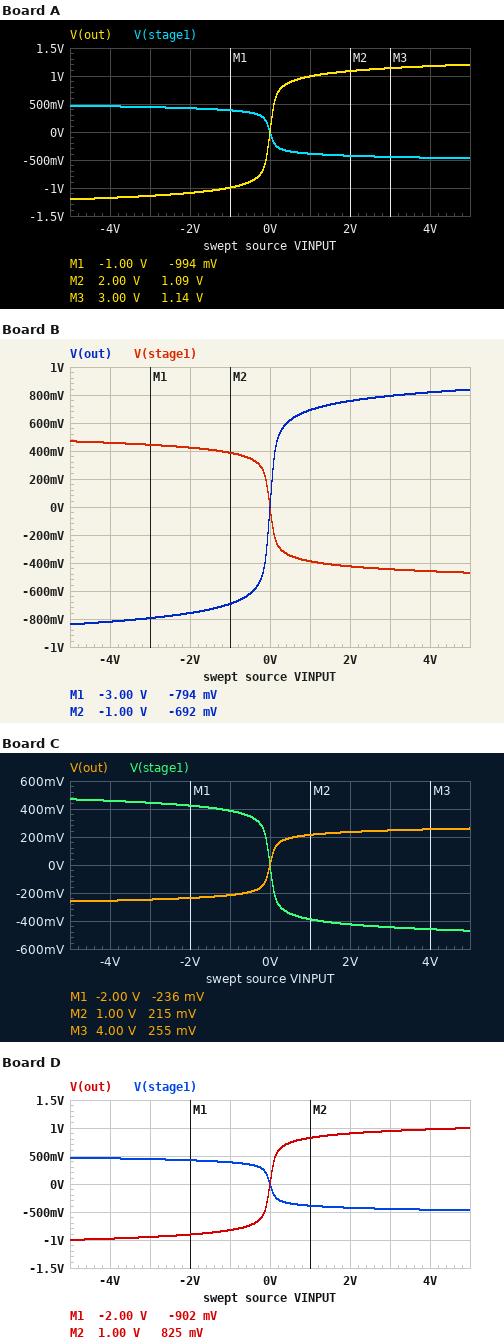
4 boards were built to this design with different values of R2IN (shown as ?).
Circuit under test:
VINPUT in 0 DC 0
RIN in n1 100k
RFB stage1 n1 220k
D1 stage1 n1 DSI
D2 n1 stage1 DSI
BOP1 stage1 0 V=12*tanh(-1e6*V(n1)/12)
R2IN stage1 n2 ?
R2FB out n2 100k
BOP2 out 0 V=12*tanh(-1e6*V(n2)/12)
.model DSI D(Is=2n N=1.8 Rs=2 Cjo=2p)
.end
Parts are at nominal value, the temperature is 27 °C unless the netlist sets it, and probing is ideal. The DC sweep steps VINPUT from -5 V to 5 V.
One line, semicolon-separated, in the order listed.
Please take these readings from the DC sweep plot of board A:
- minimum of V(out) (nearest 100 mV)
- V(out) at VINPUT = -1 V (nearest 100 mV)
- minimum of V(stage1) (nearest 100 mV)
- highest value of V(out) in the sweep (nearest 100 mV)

-1.2 V; -1.0 V; -500 mV; 1.2 V
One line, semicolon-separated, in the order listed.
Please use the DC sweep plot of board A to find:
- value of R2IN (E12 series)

39 kΩ
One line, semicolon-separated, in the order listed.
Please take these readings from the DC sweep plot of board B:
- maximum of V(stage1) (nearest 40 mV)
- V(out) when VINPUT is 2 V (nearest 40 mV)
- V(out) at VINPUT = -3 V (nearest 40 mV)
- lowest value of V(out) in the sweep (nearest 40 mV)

480 mV; 760 mV; -800 mV; -840 mV
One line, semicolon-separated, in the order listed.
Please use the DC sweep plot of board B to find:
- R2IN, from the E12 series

56 kΩ
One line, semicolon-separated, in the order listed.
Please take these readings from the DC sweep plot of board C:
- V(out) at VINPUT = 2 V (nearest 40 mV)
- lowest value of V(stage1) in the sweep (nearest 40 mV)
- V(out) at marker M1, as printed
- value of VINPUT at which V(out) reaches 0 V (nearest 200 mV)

240 mV; -480 mV; -236 mV; 0 V
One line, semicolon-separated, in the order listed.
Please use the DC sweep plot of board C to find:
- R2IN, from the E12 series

180 kΩ
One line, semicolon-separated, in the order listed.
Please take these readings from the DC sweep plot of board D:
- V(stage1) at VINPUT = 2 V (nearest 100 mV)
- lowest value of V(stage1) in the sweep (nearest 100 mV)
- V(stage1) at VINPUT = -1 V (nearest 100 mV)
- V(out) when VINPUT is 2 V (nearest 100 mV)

-400 mV; -500 mV; 400 mV; 900 mV
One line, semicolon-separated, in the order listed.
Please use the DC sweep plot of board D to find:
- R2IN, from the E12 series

47 kΩ
